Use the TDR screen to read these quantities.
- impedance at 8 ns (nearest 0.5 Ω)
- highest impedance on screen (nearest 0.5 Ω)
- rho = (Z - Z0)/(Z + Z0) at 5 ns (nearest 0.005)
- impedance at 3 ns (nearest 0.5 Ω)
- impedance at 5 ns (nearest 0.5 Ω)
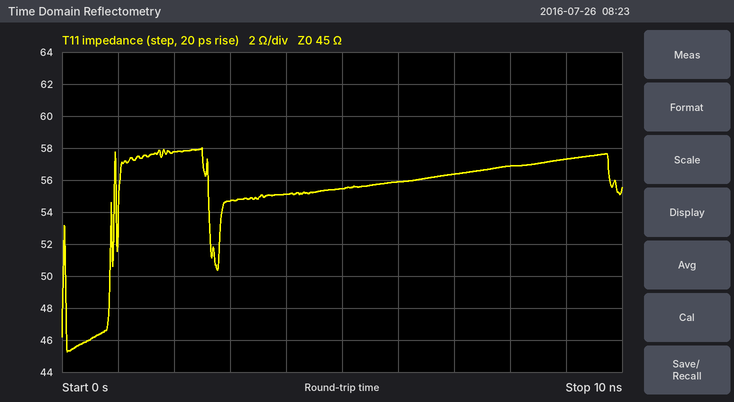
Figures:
57.0 Ω
58.0 Ω
+0.105
54.5 Ω
55.5 Ω
